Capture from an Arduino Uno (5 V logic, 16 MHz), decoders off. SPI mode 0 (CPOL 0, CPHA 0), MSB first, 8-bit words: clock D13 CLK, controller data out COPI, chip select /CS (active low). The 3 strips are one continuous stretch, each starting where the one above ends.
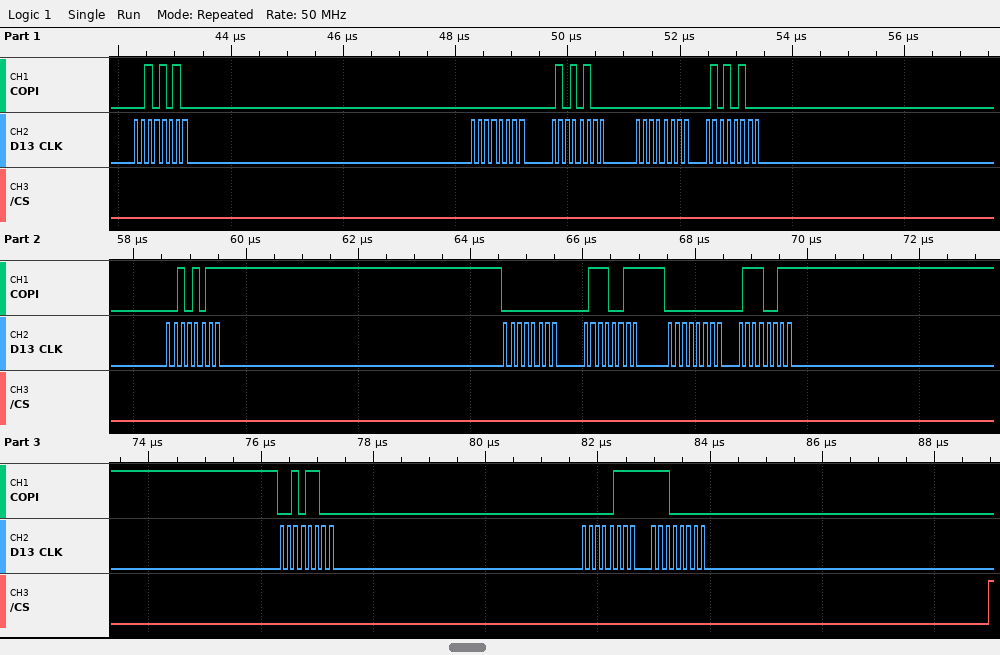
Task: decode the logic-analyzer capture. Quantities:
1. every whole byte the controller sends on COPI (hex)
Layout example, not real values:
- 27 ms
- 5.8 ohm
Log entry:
- 2A 00 54 00 54 2B 00 73 00 73 2C 07 E0
